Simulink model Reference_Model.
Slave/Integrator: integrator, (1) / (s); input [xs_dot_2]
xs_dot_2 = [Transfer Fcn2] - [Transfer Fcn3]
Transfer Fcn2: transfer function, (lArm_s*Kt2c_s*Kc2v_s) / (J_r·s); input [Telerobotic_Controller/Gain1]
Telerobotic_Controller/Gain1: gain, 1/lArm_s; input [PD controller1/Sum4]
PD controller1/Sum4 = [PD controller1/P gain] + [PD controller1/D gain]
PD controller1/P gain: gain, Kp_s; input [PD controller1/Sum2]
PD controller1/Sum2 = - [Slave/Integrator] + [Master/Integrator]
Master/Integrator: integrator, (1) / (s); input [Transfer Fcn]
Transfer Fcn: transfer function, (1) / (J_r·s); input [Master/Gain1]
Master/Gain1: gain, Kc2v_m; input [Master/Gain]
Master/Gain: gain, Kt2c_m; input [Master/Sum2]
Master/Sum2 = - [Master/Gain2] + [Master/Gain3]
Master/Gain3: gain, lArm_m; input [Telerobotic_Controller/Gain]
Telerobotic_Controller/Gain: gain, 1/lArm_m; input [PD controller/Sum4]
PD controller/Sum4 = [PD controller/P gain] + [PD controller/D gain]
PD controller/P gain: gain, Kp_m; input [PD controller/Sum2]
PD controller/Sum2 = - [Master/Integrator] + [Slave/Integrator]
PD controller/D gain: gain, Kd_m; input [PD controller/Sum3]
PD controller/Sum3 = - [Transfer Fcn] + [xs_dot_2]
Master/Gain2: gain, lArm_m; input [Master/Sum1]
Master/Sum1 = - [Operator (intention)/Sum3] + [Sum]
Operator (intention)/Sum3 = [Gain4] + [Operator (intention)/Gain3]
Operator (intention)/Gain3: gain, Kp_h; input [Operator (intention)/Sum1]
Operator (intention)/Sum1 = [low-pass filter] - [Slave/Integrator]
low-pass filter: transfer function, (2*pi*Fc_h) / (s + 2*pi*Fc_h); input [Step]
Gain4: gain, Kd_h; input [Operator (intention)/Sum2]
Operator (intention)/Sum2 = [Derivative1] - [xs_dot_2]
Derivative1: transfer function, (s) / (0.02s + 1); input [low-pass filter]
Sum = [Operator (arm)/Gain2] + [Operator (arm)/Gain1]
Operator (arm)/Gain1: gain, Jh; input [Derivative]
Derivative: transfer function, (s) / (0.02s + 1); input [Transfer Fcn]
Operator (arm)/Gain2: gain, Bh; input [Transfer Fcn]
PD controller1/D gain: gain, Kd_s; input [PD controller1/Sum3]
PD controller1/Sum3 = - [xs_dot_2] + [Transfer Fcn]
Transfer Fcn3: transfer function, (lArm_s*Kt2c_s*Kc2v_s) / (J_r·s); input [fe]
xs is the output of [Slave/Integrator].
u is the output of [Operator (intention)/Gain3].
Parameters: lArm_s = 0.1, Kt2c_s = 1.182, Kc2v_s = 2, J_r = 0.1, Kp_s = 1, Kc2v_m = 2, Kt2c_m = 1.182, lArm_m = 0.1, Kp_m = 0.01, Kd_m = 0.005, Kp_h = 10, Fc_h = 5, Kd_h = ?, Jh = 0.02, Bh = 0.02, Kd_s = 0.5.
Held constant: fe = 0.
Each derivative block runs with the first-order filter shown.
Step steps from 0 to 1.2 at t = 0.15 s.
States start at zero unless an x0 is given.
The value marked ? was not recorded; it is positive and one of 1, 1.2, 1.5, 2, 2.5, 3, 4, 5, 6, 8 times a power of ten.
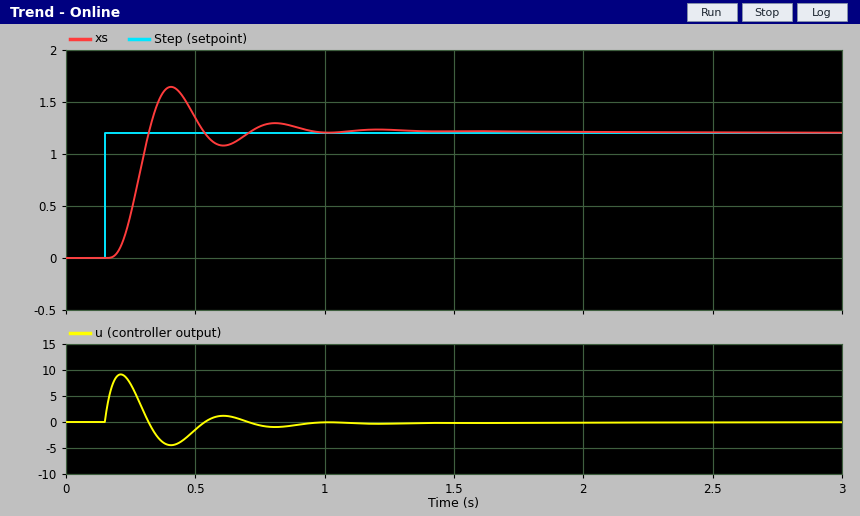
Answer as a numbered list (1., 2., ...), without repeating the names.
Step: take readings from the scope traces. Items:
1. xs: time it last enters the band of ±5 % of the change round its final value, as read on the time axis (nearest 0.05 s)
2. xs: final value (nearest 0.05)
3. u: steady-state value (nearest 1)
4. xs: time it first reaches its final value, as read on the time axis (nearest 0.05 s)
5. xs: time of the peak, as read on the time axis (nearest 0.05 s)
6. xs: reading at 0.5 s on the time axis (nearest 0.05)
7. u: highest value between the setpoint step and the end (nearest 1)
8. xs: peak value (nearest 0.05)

1. 0.90 s
2. 1.20
3. 0
4. 0.30 s
5. 0.40 s
6. 1.35
7. 9
8. 1.65
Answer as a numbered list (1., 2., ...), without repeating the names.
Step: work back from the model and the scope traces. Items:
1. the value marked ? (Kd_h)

1. 10
